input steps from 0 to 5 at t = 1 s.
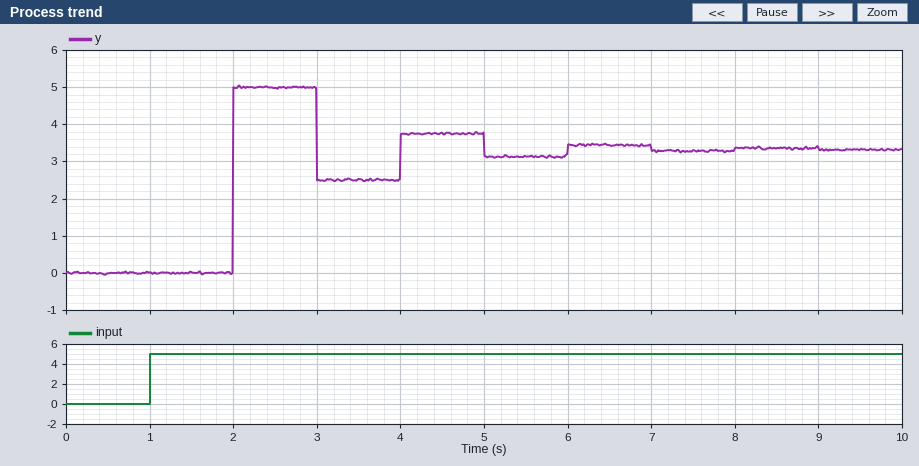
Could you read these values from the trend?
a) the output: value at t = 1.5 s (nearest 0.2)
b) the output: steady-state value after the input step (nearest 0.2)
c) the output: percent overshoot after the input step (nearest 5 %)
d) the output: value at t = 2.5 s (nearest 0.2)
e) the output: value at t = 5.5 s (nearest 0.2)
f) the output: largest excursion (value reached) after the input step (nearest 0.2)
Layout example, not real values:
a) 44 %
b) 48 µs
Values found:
a) 0.0
b) 3.4
c) 50 %
d) 5.0
e) 3.2
f) 5.0
